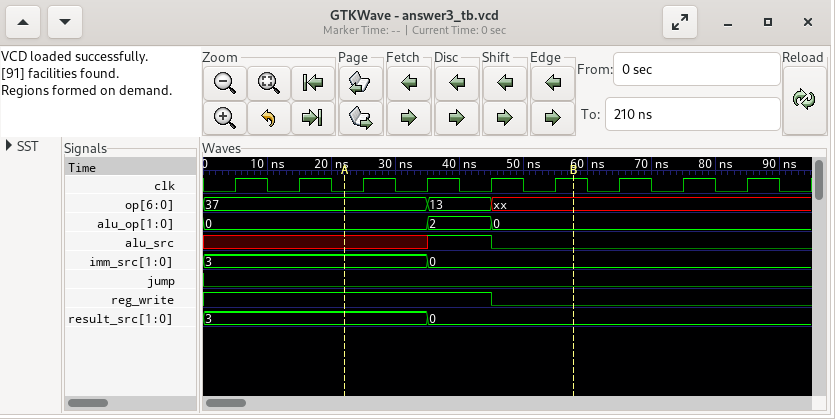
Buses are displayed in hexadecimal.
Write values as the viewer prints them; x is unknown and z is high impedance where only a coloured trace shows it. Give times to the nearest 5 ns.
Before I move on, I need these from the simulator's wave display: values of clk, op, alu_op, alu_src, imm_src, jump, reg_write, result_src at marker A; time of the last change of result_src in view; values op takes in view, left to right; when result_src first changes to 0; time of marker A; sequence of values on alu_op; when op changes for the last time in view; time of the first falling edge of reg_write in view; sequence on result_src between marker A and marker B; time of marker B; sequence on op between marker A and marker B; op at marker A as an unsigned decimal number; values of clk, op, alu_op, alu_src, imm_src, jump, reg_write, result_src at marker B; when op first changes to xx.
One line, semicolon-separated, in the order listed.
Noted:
clk=0, op=37, alu_op=0, alu_src=x, imm_src=3, jump=0, reg_write=1, result_src=3; 35 ns; 37, 13, xx; 35 ns; 20 ns; 0, 2, 0; 45 ns; 45 ns; 3, 0; 60 ns; 37, 13, xx; 55; clk=1, op=xx, alu_op=0, alu_src=0, imm_src=0, jump=0, reg_write=0, result_src=0; 45 ns
